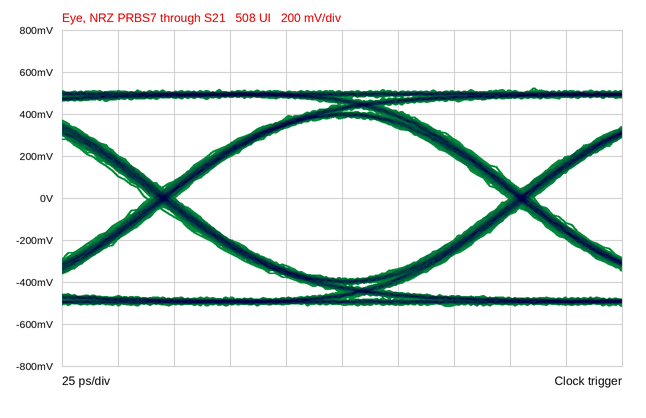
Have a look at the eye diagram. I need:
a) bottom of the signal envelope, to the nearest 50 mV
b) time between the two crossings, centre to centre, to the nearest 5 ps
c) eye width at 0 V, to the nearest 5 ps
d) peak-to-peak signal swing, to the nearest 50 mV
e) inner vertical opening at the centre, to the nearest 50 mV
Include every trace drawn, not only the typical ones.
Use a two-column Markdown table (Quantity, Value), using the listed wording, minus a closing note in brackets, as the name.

| Quantity | Value |
|---|---|
| bottom of the signal envelope, to the nearest 50 mV | -500 mV |
| time between the two crossings, centre to centre, to the nearest 5 ps | 160 ps |
| eye width at 0 V, to the nearest 5 ps | 150 ps |
| peak-to-peak signal swing, to the nearest 50 mV | 1.05 V |
| inner vertical opening at the centre, to the nearest 50 mV | 750 mV |
